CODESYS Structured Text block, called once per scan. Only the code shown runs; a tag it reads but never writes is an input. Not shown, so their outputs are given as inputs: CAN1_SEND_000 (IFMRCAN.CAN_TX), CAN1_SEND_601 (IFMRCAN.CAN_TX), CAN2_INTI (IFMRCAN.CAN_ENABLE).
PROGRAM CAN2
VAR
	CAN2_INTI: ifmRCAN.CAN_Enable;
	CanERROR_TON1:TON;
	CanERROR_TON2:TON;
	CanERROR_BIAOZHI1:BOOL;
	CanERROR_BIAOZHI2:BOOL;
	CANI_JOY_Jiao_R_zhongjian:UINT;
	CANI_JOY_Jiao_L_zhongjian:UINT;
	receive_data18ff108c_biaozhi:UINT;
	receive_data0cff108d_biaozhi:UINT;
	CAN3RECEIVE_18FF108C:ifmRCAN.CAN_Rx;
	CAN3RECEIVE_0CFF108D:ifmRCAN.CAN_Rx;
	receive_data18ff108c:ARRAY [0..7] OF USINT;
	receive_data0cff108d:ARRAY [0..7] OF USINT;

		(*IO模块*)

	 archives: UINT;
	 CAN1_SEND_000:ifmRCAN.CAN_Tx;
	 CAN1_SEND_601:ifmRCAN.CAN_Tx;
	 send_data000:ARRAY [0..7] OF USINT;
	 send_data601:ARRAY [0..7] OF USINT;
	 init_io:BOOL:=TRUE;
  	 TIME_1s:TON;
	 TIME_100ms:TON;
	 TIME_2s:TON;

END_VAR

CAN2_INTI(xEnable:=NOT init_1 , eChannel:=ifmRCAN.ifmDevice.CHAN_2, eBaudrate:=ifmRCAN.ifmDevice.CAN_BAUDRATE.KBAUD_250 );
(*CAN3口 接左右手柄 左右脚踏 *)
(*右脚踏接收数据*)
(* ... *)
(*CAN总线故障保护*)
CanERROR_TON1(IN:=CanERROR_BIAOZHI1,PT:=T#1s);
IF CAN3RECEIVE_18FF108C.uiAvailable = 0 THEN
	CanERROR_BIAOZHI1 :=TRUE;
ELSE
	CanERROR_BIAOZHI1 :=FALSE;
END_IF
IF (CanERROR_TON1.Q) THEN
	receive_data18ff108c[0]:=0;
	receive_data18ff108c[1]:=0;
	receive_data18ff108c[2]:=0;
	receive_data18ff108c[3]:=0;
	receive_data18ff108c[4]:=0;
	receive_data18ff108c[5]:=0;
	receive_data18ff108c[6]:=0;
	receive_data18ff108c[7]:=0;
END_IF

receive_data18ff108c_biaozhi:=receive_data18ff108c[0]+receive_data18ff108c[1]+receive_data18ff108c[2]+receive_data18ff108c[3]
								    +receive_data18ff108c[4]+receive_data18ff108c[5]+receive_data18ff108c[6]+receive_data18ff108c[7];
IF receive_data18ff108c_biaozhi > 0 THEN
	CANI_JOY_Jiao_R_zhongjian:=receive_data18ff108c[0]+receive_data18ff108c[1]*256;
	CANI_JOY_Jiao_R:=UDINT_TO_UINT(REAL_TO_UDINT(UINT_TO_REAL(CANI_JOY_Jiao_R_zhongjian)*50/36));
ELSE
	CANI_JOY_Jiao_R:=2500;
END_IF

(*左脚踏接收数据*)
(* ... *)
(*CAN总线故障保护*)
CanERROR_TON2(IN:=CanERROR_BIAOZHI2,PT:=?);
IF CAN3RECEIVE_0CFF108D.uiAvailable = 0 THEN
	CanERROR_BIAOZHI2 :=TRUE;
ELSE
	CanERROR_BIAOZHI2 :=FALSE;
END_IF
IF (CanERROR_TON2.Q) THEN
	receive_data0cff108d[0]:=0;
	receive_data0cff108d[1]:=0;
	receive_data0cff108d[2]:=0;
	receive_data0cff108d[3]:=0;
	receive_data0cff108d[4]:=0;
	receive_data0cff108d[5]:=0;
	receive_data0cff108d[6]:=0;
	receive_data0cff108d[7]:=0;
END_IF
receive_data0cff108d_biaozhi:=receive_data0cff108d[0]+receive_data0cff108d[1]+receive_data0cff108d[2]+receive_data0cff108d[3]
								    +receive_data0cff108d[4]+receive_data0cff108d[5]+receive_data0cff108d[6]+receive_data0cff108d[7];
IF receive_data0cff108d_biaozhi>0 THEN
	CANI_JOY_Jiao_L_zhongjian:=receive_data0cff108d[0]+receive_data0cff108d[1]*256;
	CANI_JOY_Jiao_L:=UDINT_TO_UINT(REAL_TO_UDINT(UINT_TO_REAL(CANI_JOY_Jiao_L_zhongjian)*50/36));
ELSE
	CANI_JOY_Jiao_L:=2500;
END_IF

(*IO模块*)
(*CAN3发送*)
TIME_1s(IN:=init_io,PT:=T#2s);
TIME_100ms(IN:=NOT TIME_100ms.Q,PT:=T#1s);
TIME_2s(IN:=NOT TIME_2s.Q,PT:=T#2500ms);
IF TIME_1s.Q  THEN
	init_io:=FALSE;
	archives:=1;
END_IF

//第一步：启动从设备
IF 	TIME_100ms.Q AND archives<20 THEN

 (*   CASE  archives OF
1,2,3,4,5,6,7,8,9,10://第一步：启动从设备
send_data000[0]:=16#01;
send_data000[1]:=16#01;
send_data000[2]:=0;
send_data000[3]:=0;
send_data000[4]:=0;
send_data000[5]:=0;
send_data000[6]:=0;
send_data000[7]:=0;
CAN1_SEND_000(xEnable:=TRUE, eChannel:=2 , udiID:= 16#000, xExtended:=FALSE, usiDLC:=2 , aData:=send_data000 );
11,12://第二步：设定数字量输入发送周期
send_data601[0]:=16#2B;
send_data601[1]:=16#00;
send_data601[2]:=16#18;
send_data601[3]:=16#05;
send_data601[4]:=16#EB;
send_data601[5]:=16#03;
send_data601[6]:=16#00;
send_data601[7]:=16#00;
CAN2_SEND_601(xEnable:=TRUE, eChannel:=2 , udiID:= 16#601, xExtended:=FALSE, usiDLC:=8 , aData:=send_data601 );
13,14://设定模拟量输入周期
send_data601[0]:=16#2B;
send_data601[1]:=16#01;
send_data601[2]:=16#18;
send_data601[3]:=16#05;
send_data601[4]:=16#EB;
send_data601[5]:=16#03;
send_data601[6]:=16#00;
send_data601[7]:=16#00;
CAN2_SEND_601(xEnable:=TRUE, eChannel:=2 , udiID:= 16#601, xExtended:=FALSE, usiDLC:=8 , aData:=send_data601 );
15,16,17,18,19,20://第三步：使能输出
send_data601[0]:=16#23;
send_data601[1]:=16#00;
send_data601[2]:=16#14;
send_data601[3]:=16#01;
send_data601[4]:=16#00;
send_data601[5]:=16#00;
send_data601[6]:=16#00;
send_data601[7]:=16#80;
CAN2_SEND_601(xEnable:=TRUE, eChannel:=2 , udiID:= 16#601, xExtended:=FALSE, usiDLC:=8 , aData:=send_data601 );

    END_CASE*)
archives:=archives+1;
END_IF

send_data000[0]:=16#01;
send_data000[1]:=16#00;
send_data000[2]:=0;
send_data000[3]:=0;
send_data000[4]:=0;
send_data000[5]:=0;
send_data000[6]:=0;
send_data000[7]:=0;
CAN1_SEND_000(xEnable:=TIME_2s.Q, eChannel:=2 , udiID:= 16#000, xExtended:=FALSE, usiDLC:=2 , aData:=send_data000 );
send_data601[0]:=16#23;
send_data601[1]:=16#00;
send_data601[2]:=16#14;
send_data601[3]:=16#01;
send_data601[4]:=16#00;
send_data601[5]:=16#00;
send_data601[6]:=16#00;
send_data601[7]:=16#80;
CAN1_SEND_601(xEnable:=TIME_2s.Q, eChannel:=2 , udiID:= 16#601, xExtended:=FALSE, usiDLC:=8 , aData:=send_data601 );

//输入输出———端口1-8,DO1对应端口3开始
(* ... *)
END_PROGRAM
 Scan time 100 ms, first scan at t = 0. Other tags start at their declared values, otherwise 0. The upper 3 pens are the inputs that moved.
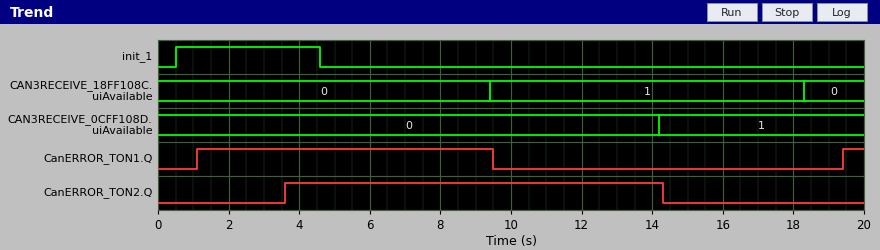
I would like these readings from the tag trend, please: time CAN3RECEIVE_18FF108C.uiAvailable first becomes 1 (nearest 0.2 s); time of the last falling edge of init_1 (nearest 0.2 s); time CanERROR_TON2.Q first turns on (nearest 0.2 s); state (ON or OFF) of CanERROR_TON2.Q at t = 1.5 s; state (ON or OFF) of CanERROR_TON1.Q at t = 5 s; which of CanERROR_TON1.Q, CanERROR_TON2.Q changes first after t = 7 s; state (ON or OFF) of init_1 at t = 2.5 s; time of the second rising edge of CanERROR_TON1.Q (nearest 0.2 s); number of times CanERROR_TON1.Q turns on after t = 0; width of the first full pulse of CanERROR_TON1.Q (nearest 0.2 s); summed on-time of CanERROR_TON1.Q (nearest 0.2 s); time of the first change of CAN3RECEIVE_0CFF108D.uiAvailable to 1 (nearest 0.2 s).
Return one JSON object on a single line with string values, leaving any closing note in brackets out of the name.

{"time CAN3RECEIVE_18FF108C.uiAvailable first becomes 1": "9.4 s", "time of the last falling edge of init_1": "4.6 s", "time CanERROR_TON2.Q first turns on": "3.6 s", "state (ON or OFF) of CanERROR_TON2.Q at t = 1.5 s": "OFF", "state (ON or OFF) of CanERROR_TON1.Q at t = 5 s": "ON", "which of CanERROR_TON1.Q, CanERROR_TON2.Q changes first after t = 7 s": "CanERROR_TON1.Q", "state (ON or OFF) of init_1 at t = 2.5 s": "ON", "time of the second rising edge of CanERROR_TON1.Q": "19.4 s", "number of times CanERROR_TON1.Q turns on after t = 0": "2", "width of the first full pulse of CanERROR_TON1.Q": "8.4 s", "summed on-time of CanERROR_TON1.Q": "9.0 s", "time of the first change of CAN3RECEIVE_0CFF108D.uiAvailable to 1": "14.2 s"}
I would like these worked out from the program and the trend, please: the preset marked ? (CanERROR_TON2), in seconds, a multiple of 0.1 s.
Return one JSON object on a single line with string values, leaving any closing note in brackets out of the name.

{"the preset marked ? (CanERROR_TON2), in seconds, a multiple of 0.1 s": "3.5 s"}
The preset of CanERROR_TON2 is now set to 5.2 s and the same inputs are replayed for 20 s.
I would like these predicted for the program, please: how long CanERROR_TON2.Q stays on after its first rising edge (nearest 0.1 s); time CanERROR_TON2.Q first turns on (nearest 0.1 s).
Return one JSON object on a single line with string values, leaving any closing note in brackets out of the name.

{"how long CanERROR_TON2.Q stays on after its first rising edge": "9.0 s", "time CanERROR_TON2.Q first turns on": "5.3 s"}
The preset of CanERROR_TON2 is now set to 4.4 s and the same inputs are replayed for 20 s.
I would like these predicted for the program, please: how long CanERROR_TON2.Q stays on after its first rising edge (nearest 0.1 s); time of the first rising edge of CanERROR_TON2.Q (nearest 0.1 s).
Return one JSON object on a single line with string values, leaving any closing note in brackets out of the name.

{"how long CanERROR_TON2.Q stays on after its first rising edge": "9.8 s", "time of the first rising edge of CanERROR_TON2.Q": "4.5 s"}
